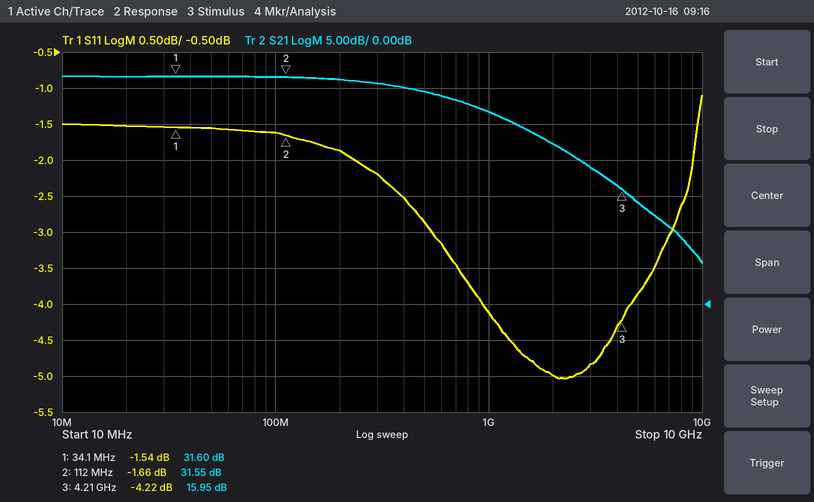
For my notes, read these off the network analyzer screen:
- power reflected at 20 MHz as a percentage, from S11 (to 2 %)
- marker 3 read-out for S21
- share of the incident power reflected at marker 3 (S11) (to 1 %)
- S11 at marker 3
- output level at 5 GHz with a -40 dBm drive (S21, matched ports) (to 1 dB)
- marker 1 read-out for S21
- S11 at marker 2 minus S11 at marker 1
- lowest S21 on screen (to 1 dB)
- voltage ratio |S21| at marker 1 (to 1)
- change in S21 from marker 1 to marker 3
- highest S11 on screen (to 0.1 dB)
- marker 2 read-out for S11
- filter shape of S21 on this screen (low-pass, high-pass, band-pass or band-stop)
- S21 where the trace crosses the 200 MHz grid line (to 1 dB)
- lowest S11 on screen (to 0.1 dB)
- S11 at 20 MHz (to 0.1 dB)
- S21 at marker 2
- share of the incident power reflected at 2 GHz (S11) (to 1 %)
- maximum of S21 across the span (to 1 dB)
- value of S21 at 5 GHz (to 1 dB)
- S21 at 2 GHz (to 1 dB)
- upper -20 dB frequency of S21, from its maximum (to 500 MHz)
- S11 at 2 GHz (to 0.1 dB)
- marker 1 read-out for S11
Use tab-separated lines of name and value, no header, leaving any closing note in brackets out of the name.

power reflected at 20 MHz as a percentage, from S11	70 %
marker 3 read-out for S21	15.95 dB
share of the incident power reflected at marker 3 (S11)	38 %
S11 at marker 3	-4.22 dB
output level at 5 GHz with a -40 dBm drive (S21, matched ports)	-26 dBm
marker 1 read-out for S21	31.60 dB
S11 at marker 2 minus S11 at marker 1	-0.12 dB
lowest S21 on screen	6 dB
voltage ratio |S21| at marker 1	38
change in S21 from marker 1 to marker 3	-15.65 dB
highest S11 on screen	-1.1 dB
marker 2 read-out for S11	-1.66 dB
filter shape of S21 on this screen	low-pass
S21 where the trace crosses the 200 MHz grid line	31 dB
lowest S11 on screen	-5.0 dB
S11 at 20 MHz	-1.5 dB
S21 at marker 2	31.55 dB
share of the incident power reflected at 2 GHz (S11)	32 %
maximum of S21 across the span	32 dB
value of S21 at 5 GHz	14 dB
S21 at 2 GHz	22 dB
upper -20 dB frequency of S21, from its maximum	6.5 GHz
S11 at 2 GHz	-5.0 dB
marker 1 read-out for S11	-1.54 dB
